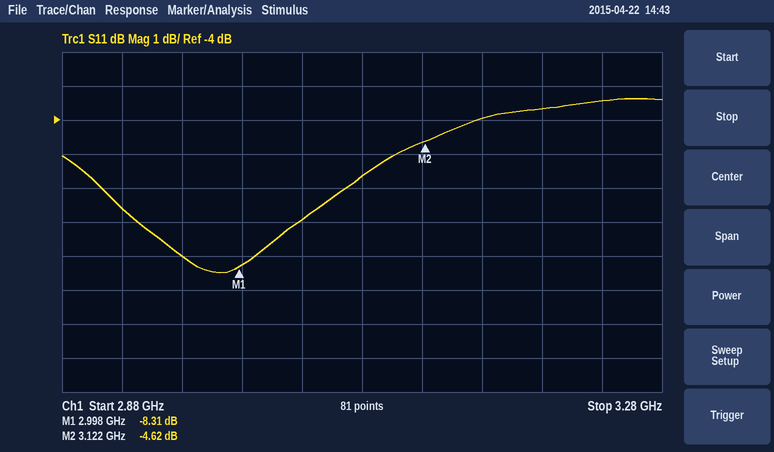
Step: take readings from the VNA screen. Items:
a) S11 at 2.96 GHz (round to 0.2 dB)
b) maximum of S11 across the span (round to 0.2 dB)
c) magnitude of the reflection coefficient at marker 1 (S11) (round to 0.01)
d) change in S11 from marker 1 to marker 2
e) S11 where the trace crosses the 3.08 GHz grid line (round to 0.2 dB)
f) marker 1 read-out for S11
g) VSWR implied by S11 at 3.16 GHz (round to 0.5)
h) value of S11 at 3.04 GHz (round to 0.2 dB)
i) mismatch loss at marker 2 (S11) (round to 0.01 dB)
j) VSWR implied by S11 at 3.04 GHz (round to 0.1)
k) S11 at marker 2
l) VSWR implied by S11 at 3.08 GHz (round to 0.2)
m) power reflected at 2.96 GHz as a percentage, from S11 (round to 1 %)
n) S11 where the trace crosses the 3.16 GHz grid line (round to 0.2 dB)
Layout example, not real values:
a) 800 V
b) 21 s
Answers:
a) -8.0 dB
b) -3.4 dB
c) 0.38
d) 3.69 dB
e) -5.6 dB
f) -8.31 dB
g) 4.5
h) -7.0 dB
i) 1.84 dB
j) 2.6
k) -4.62 dB
l) 3.2
m) 16 %
n) -4.0 dB
